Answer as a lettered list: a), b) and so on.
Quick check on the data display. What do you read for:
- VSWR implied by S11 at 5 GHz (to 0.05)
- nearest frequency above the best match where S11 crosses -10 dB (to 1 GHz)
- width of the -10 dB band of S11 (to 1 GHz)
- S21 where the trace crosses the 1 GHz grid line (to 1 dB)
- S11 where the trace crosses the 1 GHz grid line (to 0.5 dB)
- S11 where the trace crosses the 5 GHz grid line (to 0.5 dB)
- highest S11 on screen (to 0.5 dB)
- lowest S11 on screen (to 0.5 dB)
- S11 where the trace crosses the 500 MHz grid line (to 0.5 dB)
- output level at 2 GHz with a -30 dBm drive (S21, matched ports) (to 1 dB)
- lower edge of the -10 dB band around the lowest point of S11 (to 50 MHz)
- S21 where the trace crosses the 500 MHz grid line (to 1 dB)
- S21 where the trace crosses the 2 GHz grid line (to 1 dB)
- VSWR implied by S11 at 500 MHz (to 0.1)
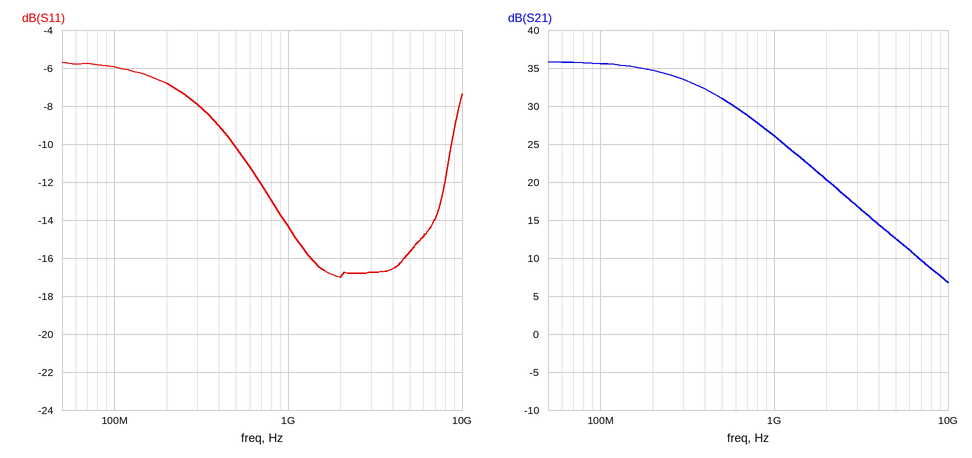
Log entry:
a) 1.40
b) 9 GHz
c) 8 GHz
d) 26 dB
e) -14.5 dB
f) -15.5 dB
g) -5.5 dB
h) -17.0 dB
i) -10.0 dB
j) -10 dBm
k) 500 MHz
l) 31 dB
m) 20 dB
n) 1.9
